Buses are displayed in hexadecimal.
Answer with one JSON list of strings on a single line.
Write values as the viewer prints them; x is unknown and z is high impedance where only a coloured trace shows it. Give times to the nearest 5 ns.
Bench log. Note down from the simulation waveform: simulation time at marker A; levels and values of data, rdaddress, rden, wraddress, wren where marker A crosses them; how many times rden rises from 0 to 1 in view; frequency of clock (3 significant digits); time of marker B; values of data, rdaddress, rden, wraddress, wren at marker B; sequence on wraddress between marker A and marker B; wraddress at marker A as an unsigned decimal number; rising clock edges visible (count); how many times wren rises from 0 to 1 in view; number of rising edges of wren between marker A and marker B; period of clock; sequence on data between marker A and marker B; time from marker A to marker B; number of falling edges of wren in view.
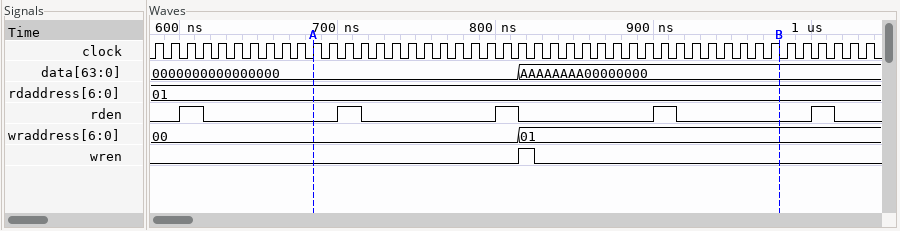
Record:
["685 ns", "data=0000000000000000, rdaddress=01, rden=0, wraddress=00, wren=0", "5", "100 MHz", "980 ns", "data=AAAAAAAA00000000, rdaddress=01, rden=0, wraddress=01, wren=0", "00, 01", "0", "46", "1", "1", "10 ns", "0000000000000000, AAAAAAAA00000000", "295 ns", "1"]
